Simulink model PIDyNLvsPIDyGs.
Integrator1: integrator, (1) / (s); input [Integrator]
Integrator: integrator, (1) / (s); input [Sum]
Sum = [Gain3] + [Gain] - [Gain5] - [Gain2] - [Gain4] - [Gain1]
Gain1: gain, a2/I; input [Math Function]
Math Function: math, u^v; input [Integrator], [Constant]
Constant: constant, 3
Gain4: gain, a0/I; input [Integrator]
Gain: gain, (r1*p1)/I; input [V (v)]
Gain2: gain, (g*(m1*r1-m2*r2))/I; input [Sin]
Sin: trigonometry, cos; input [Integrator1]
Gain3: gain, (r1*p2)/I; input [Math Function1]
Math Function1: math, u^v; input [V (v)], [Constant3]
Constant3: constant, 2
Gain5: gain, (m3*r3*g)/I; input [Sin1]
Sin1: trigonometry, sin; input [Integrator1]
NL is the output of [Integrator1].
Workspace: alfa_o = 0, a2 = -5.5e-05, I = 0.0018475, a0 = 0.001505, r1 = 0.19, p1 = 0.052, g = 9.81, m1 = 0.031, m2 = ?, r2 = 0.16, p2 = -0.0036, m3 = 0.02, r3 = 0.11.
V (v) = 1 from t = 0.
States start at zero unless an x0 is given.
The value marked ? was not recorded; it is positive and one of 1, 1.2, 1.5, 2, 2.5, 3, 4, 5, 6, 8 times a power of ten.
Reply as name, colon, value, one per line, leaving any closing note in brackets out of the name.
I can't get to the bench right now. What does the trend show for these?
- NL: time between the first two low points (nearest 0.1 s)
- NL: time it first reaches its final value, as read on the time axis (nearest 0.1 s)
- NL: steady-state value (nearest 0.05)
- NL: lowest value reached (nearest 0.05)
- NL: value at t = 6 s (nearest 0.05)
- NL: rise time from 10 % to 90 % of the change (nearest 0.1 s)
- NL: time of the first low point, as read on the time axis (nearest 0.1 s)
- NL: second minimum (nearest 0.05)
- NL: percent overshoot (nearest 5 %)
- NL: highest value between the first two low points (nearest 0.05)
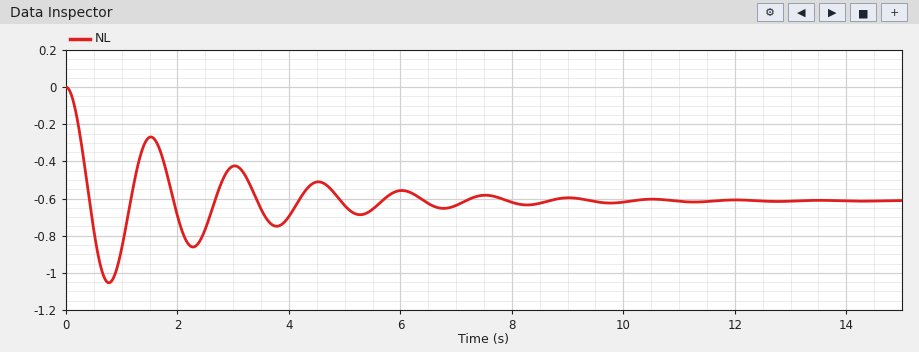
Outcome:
NL: time between the first two low points: 1.5 s
NL: time it first reaches its final value, as read on the time axis: 0.4 s
NL: steady-state value: -0.60
NL: lowest value reached: -1.05
NL: value at t = 6 s: -0.55
NL: rise time from 10 % to 90 % of the change: 0.3 s
NL: time of the first low point, as read on the time axis: 0.8 s
NL: second minimum: -0.85
NL: percent overshoot: 70 %
NL: highest value between the first two low points: -0.25
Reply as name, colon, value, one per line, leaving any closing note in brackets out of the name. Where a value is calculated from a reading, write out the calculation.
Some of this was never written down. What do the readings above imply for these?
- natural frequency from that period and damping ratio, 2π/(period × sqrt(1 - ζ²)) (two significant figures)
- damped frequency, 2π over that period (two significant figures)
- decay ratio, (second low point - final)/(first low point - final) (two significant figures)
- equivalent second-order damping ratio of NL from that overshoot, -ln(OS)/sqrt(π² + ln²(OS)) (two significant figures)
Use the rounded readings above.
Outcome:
natural frequency from that period and damping ratio, 2π/(period × sqrt(1 - ζ²)): 2π / (1.5 × sqrt(1 - 0.11²)) = 4.2 rad/s
damped frequency, 2π over that period: 2π / 1.5 = 4.2 rad/s
decay ratio, (second low point - final)/(first low point - final): (-0.85 - (-0.6)) / (-1.05 - (-0.6)) = 0.56
equivalent second-order damping ratio of NL from that overshoot, -ln(OS)/sqrt(π² + ln²(OS)): ln(0.7) = -0.357; 0.357 / sqrt(9.870 + 0.127) = 0.11
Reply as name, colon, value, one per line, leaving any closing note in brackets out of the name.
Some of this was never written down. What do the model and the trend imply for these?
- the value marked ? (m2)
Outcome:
the value marked ?: 0.02
